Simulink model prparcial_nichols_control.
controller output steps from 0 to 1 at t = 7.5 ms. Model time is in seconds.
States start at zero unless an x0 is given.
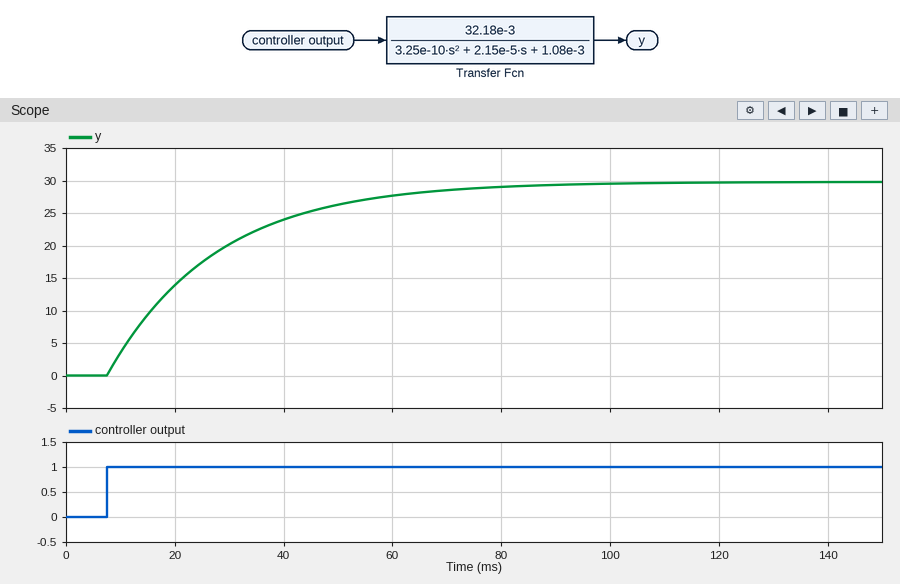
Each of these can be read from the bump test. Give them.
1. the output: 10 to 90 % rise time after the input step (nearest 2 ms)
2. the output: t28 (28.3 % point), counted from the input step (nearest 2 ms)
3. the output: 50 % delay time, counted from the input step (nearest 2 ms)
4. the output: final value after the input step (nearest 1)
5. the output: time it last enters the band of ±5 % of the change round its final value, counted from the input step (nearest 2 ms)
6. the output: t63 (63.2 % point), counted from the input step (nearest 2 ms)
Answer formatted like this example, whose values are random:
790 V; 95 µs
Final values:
44 ms; 6 ms; 14 ms; 30; 60 ms; 20 ms
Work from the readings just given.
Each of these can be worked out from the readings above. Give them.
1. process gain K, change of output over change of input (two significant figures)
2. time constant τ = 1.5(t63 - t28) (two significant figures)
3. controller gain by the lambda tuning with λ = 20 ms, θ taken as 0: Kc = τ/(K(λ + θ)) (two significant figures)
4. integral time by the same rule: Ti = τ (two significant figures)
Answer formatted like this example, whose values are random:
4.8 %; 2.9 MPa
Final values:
30; 21 ms; 0.035; 21 ms
